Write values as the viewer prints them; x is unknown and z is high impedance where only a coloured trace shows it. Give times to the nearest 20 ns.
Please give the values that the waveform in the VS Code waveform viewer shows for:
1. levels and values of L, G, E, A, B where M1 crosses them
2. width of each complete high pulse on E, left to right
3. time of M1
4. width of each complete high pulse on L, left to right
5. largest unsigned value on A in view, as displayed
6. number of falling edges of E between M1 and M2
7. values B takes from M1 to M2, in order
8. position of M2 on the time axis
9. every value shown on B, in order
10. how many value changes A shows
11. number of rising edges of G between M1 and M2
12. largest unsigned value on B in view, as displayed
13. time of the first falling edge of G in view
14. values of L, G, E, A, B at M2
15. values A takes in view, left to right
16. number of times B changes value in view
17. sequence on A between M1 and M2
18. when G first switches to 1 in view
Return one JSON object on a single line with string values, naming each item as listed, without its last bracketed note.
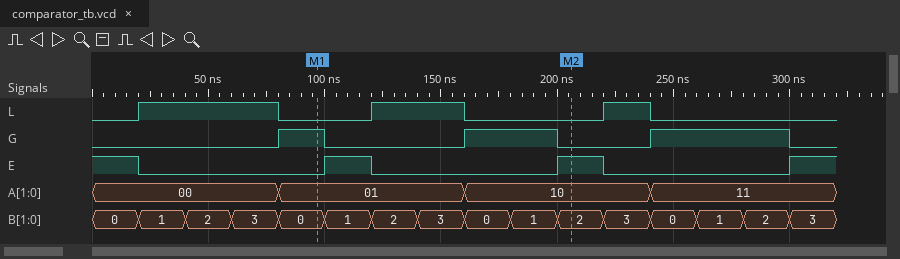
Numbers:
{"levels and values of L, G, E, A, B where M1 crosses them": "L=0, G=1, E=0, A=01, B=0", "width of each complete high pulse on E, left to right": "20 ns, 20 ns", "time of M1": "100 ns", "width of each complete high pulse on L, left to right": "60 ns, 40 ns, 20 ns", "largest unsigned value on A in view, as displayed": "11", "number of falling edges of E between M1 and M2": "1", "values B takes from M1 to M2, in order": "0, 1, 2, 3, 0, 1, 2", "position of M2 on the time axis": "200 ns", "every value shown on B, in order": "0, 1, 2, 3, 0, 1, 2, 3, 0, 1, 2, 3, 0, 1, 2, 3", "how many value changes A shows": "3", "number of rising edges of G between M1 and M2": "1", "largest unsigned value on B in view, as displayed": "3", "time of the first falling edge of G in view": "100 ns", "values of L, G, E, A, B at M2": "L=0, G=0, E=1, A=10, B=2", "values A takes in view, left to right": "00, 01, 10, 11", "number of times B changes value in view": "15", "sequence on A between M1 and M2": "01, 10", "when G first switches to 1 in view": "80 ns"}
